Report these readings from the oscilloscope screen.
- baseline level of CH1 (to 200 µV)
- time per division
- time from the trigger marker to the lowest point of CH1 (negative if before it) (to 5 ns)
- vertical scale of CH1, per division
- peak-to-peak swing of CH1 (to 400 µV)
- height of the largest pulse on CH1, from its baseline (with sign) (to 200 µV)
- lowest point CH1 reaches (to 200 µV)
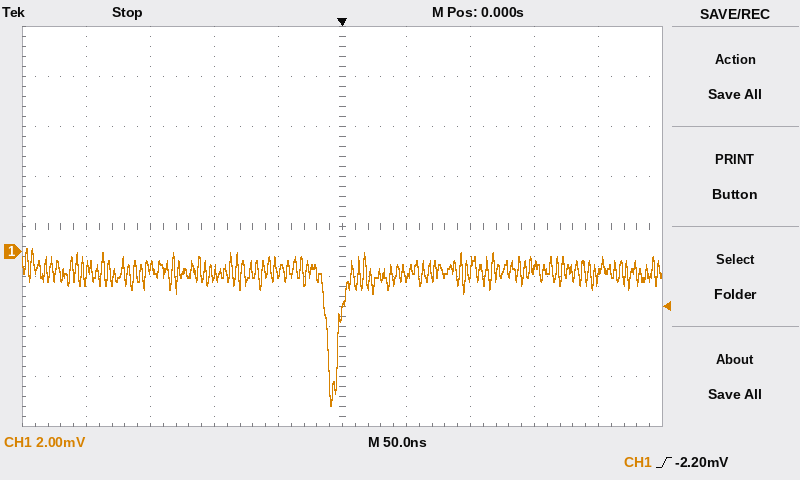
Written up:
-800 µV
50 ns
-10 ns
2 mV
6.4 mV
-5.4 mV
-6.2 mV
